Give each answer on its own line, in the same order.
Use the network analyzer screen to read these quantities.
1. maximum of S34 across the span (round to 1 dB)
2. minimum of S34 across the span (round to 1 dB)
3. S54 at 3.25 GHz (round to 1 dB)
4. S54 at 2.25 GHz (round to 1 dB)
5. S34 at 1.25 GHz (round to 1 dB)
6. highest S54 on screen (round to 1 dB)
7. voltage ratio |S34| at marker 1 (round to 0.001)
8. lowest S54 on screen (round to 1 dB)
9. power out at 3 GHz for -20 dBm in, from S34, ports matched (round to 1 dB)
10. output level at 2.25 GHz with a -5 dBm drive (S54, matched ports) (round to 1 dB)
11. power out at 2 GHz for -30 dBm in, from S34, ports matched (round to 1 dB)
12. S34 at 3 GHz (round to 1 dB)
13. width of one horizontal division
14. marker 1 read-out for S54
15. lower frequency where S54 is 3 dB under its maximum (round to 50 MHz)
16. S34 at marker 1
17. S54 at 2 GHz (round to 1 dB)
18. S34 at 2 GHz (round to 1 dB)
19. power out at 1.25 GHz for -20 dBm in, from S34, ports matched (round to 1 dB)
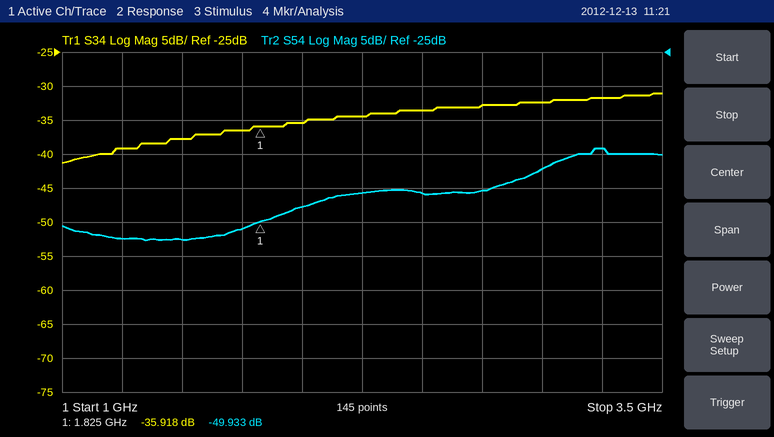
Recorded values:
-31 dB
-41 dB
-39 dB
-46 dB
-39 dB
-39 dB
0.016
-53 dB
-52 dBm
-51 dBm
-65 dBm
-32 dB
250 MHz
-49.933 dB
3.00 GHz
-35.918 dB
-48 dB
-35 dB
-59 dBm
